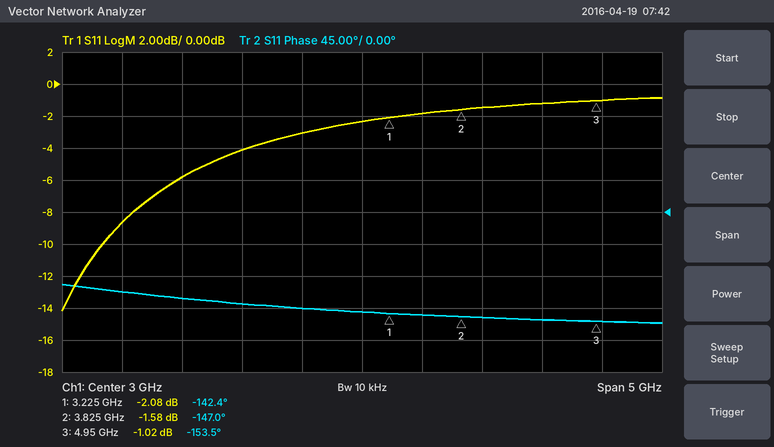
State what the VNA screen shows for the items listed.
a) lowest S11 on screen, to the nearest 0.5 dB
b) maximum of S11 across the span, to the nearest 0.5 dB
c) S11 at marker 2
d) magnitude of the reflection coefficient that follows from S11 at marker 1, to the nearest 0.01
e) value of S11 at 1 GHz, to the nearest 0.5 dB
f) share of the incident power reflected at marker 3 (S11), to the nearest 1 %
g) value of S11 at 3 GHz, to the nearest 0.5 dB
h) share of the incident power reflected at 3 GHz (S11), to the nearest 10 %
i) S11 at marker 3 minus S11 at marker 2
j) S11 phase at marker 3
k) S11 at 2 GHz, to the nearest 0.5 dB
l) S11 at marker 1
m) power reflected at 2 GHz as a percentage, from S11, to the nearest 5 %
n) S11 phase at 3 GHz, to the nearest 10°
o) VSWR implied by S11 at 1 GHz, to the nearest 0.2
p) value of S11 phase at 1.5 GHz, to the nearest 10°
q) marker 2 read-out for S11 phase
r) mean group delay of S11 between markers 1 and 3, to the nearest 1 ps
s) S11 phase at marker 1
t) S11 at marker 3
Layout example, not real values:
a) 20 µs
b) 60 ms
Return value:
a) -14.0 dB
b) -1.0 dB
c) -1.58 dB
d) 0.79
e) -8.5 dB
f) 79 %
g) -2.5 dB
h) 60 %
i) 0.56 dB
j) -153.5°
k) -4.0 dB
l) -2.08 dB
m) 40 %
n) -140°
o) 2.2
p) -120°
q) -147.0°
r) 18 ps
s) -142.4°
t) -1.02 dB
